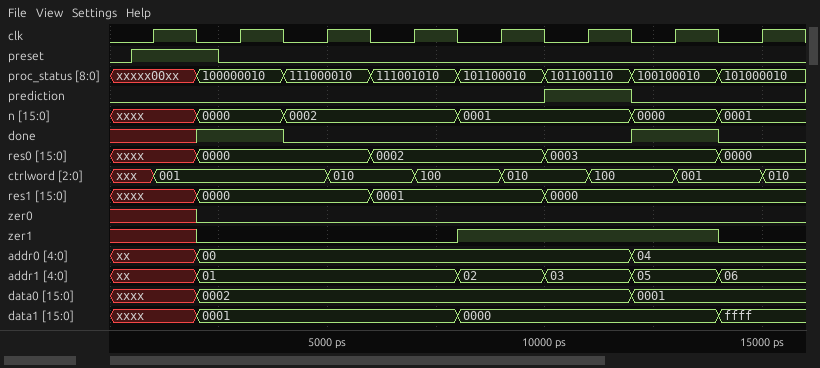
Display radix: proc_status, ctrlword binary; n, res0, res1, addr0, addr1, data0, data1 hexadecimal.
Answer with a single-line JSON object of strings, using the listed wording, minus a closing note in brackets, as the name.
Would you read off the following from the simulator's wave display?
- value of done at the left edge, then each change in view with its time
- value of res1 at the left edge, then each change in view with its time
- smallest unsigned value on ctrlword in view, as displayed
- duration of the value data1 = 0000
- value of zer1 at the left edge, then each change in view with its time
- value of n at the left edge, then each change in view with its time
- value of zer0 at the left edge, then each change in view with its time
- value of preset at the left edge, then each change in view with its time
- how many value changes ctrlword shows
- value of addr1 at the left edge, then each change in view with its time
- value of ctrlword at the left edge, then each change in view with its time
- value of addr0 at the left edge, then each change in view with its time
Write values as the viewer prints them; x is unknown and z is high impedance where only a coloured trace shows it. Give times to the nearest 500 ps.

{"value of done at the left edge, then each change in view with its time": "x, 1 at 2000 ps, 0 at 4000 ps, 1 at 12000 ps, 0 at 14000 ps", "value of res1 at the left edge, then each change in view with its time": "xxxx, 0000 at 2000 ps, 0001 at 6000 ps, 0000 at 10000 ps", "smallest unsigned value on ctrlword in view, as displayed": "001", "duration of the value data1 = 0000": "6000 ps", "value of zer1 at the left edge, then each change in view with its time": "x, 0 at 2000 ps, 1 at 8000 ps, 0 at 14000 ps", "value of n at the left edge, then each change in view with its time": "xxxx, 0000 at 2000 ps, 0002 at 4000 ps, 0001 at 8000 ps, 0000 at 12000 ps, 0001 at 14000 ps", "value of zer0 at the left edge, then each change in view with its time": "x, 0 at 2000 ps", "value of preset at the left edge, then each change in view with its time": "0, 1 at 500 ps, 0 at 2500 ps", "how many value changes ctrlword shows": "7", "value of addr1 at the left edge, then each change in view with its time": "xx, 01 at 2000 ps, 02 at 8000 ps, 03 at 10000 ps, 05 at 12000 ps, 06 at 14000 ps", "value of ctrlword at the left edge, then each change in view with its time": "xxx, 001 at 1000 ps, 010 at 5000 ps, 100 at 7000 ps, 010 at 9000 ps, 100 at 11000 ps, 001 at 13000 ps, 010 at 15000 ps", "value of addr0 at the left edge, then each change in view with its time": "xx, 00 at 2000 ps, 04 at 12000 ps"}
